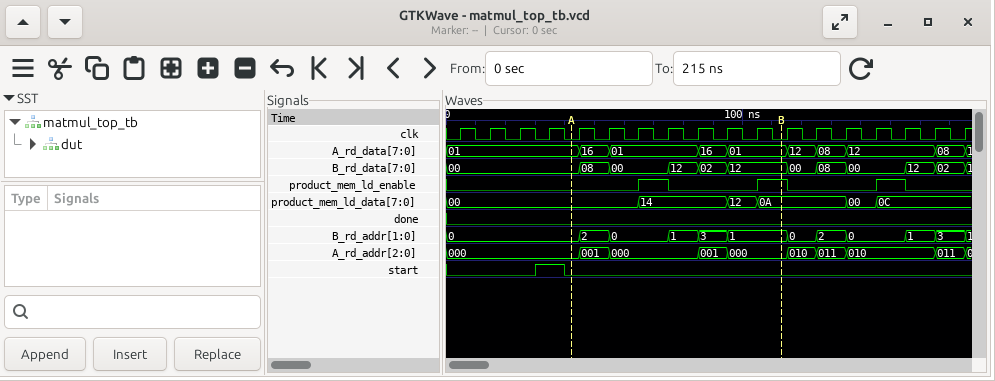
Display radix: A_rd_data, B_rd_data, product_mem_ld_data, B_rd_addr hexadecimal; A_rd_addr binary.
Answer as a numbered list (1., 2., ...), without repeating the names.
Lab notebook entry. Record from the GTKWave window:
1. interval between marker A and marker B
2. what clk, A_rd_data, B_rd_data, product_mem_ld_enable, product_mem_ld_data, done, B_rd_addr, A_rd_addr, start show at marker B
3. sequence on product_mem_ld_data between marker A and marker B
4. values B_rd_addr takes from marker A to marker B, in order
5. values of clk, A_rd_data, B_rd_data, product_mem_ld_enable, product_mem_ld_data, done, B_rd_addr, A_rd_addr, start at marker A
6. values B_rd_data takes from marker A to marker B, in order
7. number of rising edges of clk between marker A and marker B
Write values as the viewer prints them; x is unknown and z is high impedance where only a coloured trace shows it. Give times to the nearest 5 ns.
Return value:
1. 70 ns
2. clk=0, A_rd_data=01, B_rd_data=12, product_mem_ld_enable=1, product_mem_ld_data=0A, done=0, B_rd_addr=1, A_rd_addr=000, start=0
3. 00, 14, 12, 0A
4. 0, 2, 0, 1, 3, 1
5. clk=0, A_rd_data=01, B_rd_data=00, product_mem_ld_enable=0, product_mem_ld_data=00, done=0, B_rd_addr=0, A_rd_addr=000, start=0
6. 00, 08, 00, 12, 02, 12
7. 7
